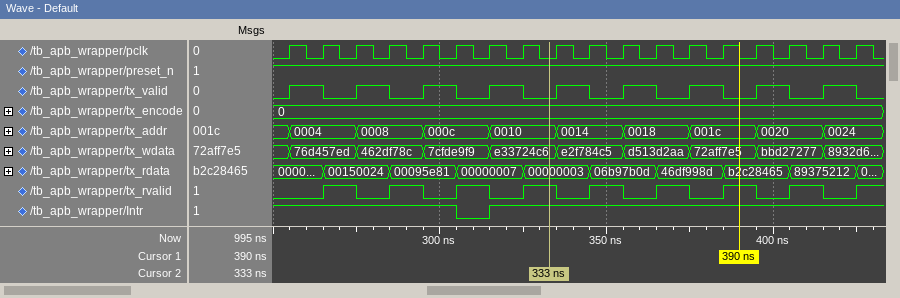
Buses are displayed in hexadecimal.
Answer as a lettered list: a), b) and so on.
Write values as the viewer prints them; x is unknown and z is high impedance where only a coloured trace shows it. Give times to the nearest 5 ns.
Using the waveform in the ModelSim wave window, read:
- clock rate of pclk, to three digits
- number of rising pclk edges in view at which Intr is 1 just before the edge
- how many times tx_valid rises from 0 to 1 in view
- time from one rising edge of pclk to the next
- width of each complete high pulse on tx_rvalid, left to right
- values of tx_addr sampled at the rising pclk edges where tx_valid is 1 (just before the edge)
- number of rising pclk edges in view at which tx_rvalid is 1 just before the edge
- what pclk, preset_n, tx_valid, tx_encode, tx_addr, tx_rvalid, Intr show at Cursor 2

a) 100 MHz
b) 17
c) 9
d) 10 ns
e) 10 ns, 10 ns, 10 ns, 10 ns, 10 ns, 10 ns, 10 ns, 10 ns
f) 0004, 0008, 000c, 0010, 0014, 0018, 001c, 0020, 0024
g) 8
h) pclk=0, preset_n=1, tx_valid=0, tx_encode=0, tx_addr=0010, tx_rvalid=1, Intr=1
